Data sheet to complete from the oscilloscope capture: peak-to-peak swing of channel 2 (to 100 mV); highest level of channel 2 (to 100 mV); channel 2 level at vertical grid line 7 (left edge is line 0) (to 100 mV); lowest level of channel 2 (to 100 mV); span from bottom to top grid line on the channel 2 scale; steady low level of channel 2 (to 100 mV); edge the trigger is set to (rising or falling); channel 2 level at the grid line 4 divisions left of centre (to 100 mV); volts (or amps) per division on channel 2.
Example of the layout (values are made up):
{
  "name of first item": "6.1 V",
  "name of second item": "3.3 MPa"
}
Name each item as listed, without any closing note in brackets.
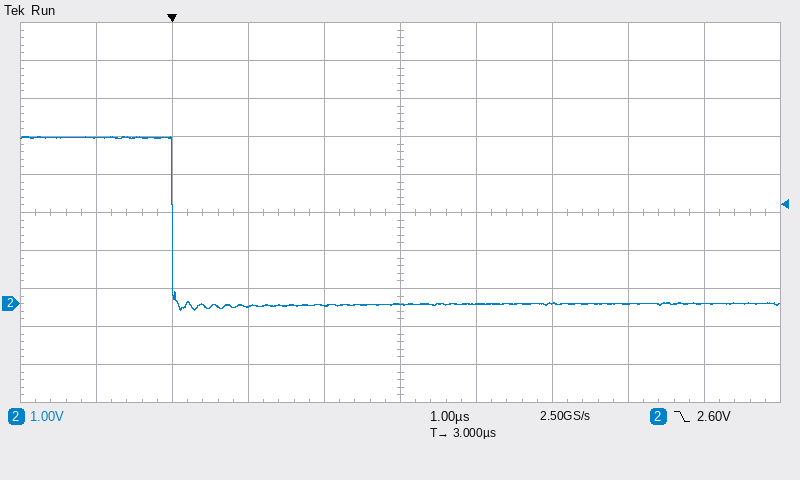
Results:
{
  "peak-to-peak swing of channel 2": "4.6 V",
  "highest level of channel 2": "4.4 V",
  "channel 2 level at vertical grid line 7 (left edge is line 0)": "0.0 V",
  "lowest level of channel 2": "-200 mV",
  "span from bottom to top grid line on the channel 2 scale": "10 V",
  "steady low level of channel 2": "0.0 V",
  "edge the trigger is set to": "falling",
  "channel 2 level at the grid line 4 divisions left of centre": "4.4 V",
  "volts (or amps) per division on channel 2": "1 V"
}
